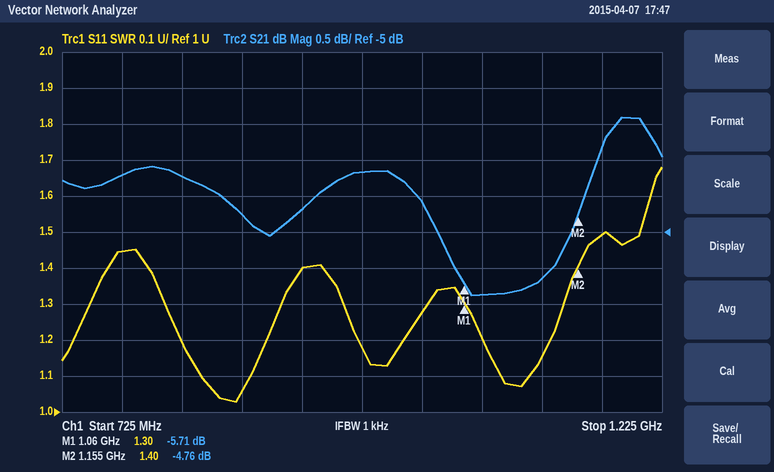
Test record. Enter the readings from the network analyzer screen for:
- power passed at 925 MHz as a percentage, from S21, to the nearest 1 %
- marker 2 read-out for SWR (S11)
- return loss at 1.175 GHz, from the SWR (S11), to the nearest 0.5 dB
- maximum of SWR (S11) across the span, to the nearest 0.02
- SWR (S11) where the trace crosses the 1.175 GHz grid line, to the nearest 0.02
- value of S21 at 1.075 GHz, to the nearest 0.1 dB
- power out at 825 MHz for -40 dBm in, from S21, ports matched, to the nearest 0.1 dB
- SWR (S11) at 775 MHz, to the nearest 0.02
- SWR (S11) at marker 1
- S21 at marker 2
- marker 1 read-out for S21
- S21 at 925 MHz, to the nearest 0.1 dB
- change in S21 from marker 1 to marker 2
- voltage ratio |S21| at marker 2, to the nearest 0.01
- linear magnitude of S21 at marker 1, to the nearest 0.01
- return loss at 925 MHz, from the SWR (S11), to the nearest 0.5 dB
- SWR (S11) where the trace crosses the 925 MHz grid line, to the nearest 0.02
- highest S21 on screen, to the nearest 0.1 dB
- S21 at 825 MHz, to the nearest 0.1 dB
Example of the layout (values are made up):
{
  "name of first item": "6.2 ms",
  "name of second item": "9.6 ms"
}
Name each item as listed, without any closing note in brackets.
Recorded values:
{
  "power passed at 925 MHz as a percentage, from S21, to the nearest 1 %": "34 %",
  "marker 2 read-out for SWR": "1.40",
  "return loss at 1.175 GHz, from the SWR (S11), to the nearest 0.5 dB": "14.0 dB",
  "maximum of SWR (S11) across the span, to the nearest 0.02": "1.68",
  "SWR (S11) where the trace crosses the 1.175 GHz grid line, to the nearest 0.02": "1.50",
  "value of S21 at 1.075 GHz, to the nearest 0.1 dB": "-5.9 dB",
  "power out at 825 MHz for -40 dBm in, from S21, ports matched, to the nearest 0.1 dB": "-44.2 dBm",
  "SWR (S11) at 775 MHz, to the nearest 0.02": "1.44",
  "SWR (S11) at marker 1": "1.30",
  "S21 at marker 2": "-4.76 dB",
  "marker 1 read-out for S21": "-5.71 dB",
  "S21 at 925 MHz, to the nearest 0.1 dB": "-4.7 dB",
  "change in S21 from marker 1 to marker 2": "0.95 dB",
  "voltage ratio |S21| at marker 2, to the nearest 0.01": "0.58",
  "linear magnitude of S21 at marker 1, to the nearest 0.01": "0.52",
  "return loss at 925 MHz, from the SWR (S11), to the nearest 0.5 dB": "15.5 dB",
  "SWR (S11) where the trace crosses the 925 MHz grid line, to the nearest 0.02": "1.40",
  "highest S21 on screen, to the nearest 0.1 dB": "-3.4 dB",
  "S21 at 825 MHz, to the nearest 0.1 dB": "-4.2 dB"
}
